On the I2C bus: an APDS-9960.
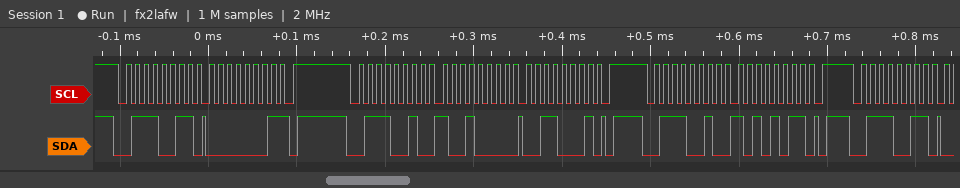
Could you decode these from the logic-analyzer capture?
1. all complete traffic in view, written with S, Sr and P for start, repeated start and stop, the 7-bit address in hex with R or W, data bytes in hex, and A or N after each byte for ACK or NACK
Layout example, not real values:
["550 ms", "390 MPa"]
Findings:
["S 39R A 01 N P S 39W A 90 A 31 A P S 39W A AB A P S 39R A"]
